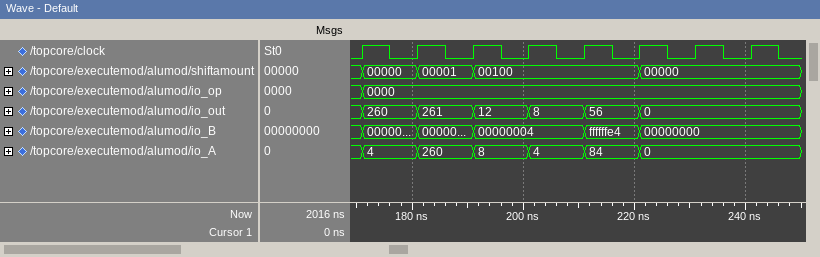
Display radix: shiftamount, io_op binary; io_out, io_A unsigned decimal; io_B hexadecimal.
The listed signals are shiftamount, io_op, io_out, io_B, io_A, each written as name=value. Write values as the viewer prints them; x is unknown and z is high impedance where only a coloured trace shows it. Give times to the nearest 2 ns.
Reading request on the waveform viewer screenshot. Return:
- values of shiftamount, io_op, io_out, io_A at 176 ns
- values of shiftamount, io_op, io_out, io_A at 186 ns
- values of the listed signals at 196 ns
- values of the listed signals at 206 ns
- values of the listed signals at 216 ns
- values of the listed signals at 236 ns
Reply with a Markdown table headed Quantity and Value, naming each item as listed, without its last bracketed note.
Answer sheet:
| Quantity | Value |
|---|---|
| values of shiftamount, io_op, io_out, io_A at 176 ns | shiftamount=00000, io_op=0000, io_out=260, io_A=4 |
| values of shiftamount, io_op, io_out, io_A at 186 ns | shiftamount=00001, io_op=0000, io_out=261, io_A=260 |
| values of the listed signals at 196 ns | shiftamount=00100, io_op=0000, io_out=12, io_B=00000004, io_A=8 |
| values of the listed signals at 206 ns | shiftamount=00100, io_op=0000, io_out=8, io_B=00000004, io_A=4 |
| values of the listed signals at 216 ns | shiftamount=00100, io_op=0000, io_out=56, io_B=ffffffe4, io_A=84 |
| values of the listed signals at 236 ns | shiftamount=00000, io_op=0000, io_out=0, io_B=00000000, io_A=0 |
